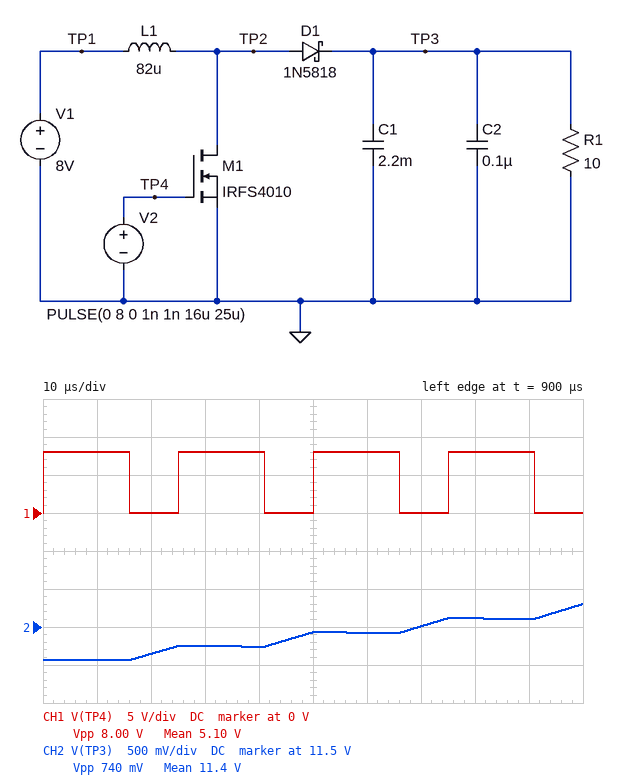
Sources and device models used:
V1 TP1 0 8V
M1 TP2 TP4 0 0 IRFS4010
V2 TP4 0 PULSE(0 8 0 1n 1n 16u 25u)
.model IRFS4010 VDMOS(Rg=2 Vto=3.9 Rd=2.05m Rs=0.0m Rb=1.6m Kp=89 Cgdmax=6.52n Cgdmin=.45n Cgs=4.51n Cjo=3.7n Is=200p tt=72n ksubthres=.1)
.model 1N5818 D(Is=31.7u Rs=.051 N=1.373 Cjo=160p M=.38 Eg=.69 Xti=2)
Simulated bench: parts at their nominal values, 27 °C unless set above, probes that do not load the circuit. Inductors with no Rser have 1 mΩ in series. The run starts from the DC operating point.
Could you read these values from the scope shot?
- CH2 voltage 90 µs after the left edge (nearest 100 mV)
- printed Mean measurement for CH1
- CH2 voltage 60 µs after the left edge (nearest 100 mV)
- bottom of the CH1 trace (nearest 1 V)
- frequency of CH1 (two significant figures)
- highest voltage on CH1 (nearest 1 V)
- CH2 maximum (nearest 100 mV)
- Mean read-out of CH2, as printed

11.6 V
5.10 V
11.4 V
0 V
40 kHz
8 V
11.8 V
11.4 V
